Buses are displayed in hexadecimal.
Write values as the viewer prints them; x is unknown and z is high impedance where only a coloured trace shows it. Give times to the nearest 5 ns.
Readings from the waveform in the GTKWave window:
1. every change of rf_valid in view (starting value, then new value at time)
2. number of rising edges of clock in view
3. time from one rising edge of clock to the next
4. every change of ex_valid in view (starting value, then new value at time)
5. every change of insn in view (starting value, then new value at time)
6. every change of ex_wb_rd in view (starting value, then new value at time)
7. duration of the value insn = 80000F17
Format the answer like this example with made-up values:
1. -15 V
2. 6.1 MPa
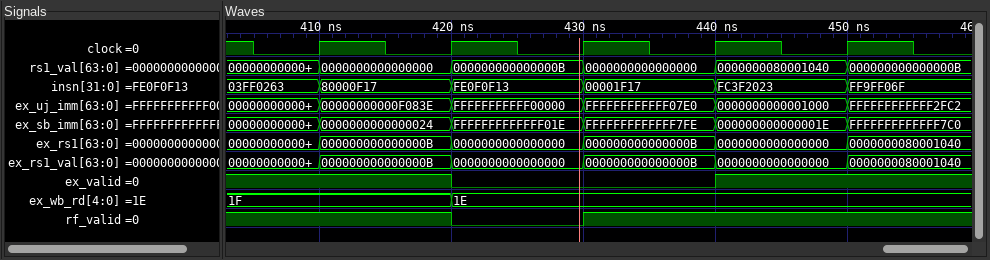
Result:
1. 1, 0 at 420 ns, 1 at 430 ns
2. 5
3. 10 ns
4. 1, 0 at 420 ns, 1 at 440 ns
5. 03FF0263, 80000F17 at 410 ns, FE0F0F13 at 420 ns, 00001F17 at 430 ns, FC3F2023 at 440 ns, FF9FF06F at 450 ns
6. 1F, 1E at 420 ns
7. 10 ns
